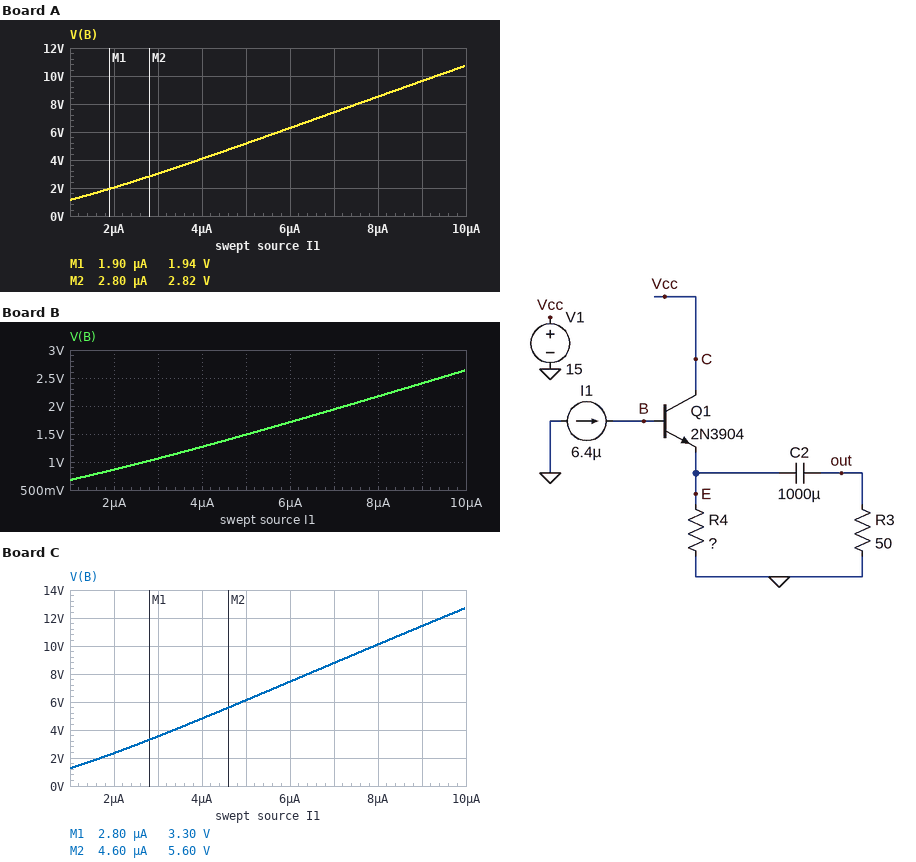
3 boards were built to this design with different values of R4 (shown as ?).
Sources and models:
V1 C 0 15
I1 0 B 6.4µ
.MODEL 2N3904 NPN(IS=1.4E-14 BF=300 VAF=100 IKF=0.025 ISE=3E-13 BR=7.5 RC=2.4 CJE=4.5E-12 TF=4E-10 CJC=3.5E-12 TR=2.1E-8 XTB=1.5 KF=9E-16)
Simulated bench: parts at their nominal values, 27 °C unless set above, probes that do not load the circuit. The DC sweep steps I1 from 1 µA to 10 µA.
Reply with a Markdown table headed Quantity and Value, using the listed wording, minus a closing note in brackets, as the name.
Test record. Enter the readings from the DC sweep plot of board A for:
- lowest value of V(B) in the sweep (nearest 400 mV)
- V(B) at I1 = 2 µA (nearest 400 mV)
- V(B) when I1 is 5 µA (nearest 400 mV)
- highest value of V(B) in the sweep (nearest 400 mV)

| Quantity | Value |
|---|---|
| lowest value of V(B) in the sweep | 1.2 V |
| V(B) at I1 = 2 µA | 2.0 V |
| V(B) when I1 is 5 µA | 5.2 V |
| highest value of V(B) in the sweep | 10.8 V |
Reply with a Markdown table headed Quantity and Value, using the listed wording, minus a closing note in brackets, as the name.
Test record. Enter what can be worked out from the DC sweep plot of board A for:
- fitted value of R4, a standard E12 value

| Quantity | Value |
|---|---|
| fitted value of R4, a standard E12 value | 8.2 kΩ |
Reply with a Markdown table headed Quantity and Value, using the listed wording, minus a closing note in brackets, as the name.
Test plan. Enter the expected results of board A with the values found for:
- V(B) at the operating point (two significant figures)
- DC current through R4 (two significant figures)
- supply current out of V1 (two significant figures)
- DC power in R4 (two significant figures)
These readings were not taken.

| Quantity | Value |
|---|---|
| V(B) at the operating point | 6.7 V |
| DC current through R4 | 740 µA |
| supply current out of V1 | 740 µA |
| DC power in R4 | 4.5 mW |
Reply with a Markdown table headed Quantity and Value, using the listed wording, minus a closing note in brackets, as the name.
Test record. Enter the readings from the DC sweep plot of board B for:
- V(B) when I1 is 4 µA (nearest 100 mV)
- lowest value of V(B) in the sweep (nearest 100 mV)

| Quantity | Value |
|---|---|
| V(B) when I1 is 4 µA | 1.3 V |
| lowest value of V(B) in the sweep | 700 mV |
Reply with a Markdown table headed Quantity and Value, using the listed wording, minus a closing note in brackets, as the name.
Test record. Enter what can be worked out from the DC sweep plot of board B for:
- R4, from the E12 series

| Quantity | Value |
|---|---|
| R4, from the E12 series | 1.5 kΩ |
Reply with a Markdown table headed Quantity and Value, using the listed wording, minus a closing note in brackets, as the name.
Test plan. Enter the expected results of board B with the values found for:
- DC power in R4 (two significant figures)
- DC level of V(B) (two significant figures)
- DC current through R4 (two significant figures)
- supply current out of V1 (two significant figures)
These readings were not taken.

| Quantity | Value |
|---|---|
| DC power in R4 | 910 µW |
| DC level of V(B) | 1.8 V |
| DC current through R4 | 780 µA |
| supply current out of V1 | 770 µA |
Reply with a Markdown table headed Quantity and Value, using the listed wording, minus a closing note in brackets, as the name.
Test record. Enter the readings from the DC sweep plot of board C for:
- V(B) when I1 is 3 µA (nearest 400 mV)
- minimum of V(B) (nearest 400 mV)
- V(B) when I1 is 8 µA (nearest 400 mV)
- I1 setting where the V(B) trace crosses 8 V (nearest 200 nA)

| Quantity | Value |
|---|---|
| V(B) when I1 is 3 µA | 3.6 V |
| minimum of V(B) | 1.2 V |
| V(B) when I1 is 8 µA | 10.0 V |
| I1 setting where the V(B) trace crosses 8 V | 6.4 µA |
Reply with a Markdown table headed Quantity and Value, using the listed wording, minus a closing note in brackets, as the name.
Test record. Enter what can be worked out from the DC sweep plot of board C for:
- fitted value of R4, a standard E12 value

| Quantity | Value |
|---|---|
| fitted value of R4, a standard E12 value | 10 kΩ |
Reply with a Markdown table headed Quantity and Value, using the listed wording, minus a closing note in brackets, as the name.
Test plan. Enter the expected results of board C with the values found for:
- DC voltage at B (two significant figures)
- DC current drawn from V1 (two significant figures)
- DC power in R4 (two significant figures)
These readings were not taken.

| Quantity | Value |
|---|---|
| DC voltage at B | 8.0 V |
| DC current drawn from V1 | 730 µA |
| DC power in R4 | 5.4 mW |
